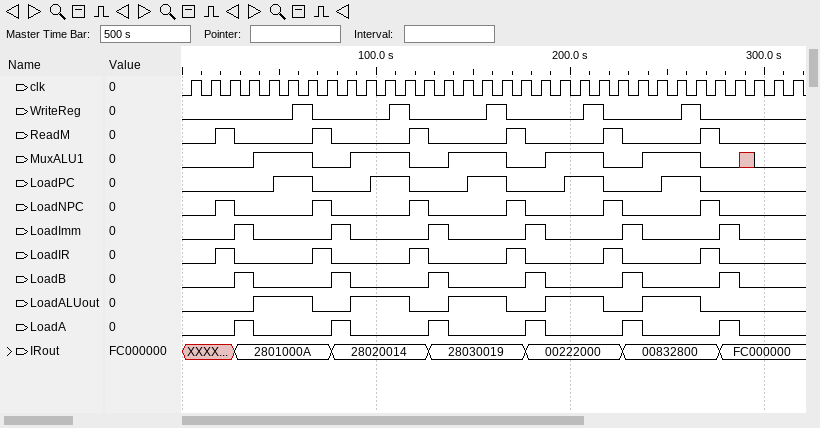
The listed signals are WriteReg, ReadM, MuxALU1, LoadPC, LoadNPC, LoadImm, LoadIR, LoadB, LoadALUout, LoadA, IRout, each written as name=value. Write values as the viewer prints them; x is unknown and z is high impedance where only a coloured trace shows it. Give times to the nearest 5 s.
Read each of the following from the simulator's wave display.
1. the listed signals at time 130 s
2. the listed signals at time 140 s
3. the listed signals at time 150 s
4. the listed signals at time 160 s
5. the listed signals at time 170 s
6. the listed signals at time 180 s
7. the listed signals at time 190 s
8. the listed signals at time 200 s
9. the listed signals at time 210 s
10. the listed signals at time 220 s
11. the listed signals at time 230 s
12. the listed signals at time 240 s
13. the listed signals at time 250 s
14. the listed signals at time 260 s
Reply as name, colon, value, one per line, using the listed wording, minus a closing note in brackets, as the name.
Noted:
the listed signals at time 130 s: WriteReg=0, ReadM=0, MuxALU1=0, LoadPC=0, LoadNPC=0, LoadImm=1, LoadIR=0, LoadB=1, LoadALUout=0, LoadA=1, IRout=28030019
the listed signals at time 140 s: WriteReg=0, ReadM=0, MuxALU1=1, LoadPC=0, LoadNPC=0, LoadImm=0, LoadIR=0, LoadB=0, LoadALUout=1, LoadA=0, IRout=28030019
the listed signals at time 150 s: WriteReg=0, ReadM=0, MuxALU1=1, LoadPC=1, LoadNPC=0, LoadImm=0, LoadIR=0, LoadB=0, LoadALUout=1, LoadA=0, IRout=28030019
the listed signals at time 160 s: WriteReg=1, ReadM=0, MuxALU1=1, LoadPC=1, LoadNPC=0, LoadImm=0, LoadIR=0, LoadB=0, LoadALUout=1, LoadA=0, IRout=28030019
the listed signals at time 170 s: WriteReg=0, ReadM=1, MuxALU1=0, LoadPC=0, LoadNPC=1, LoadImm=0, LoadIR=1, LoadB=0, LoadALUout=0, LoadA=0, IRout=28030019
the listed signals at time 180 s: WriteReg=0, ReadM=0, MuxALU1=0, LoadPC=0, LoadNPC=0, LoadImm=1, LoadIR=0, LoadB=1, LoadALUout=0, LoadA=1, IRout=00222000
the listed signals at time 190 s: WriteReg=0, ReadM=0, MuxALU1=1, LoadPC=0, LoadNPC=0, LoadImm=0, LoadIR=0, LoadB=0, LoadALUout=1, LoadA=0, IRout=00222000
the listed signals at time 200 s: WriteReg=0, ReadM=0, MuxALU1=1, LoadPC=1, LoadNPC=0, LoadImm=0, LoadIR=0, LoadB=0, LoadALUout=1, LoadA=0, IRout=00222000
the listed signals at time 210 s: WriteReg=1, ReadM=0, MuxALU1=1, LoadPC=1, LoadNPC=0, LoadImm=0, LoadIR=0, LoadB=0, LoadALUout=1, LoadA=0, IRout=00222000
the listed signals at time 220 s: WriteReg=0, ReadM=1, MuxALU1=0, LoadPC=0, LoadNPC=1, LoadImm=0, LoadIR=1, LoadB=0, LoadALUout=0, LoadA=0, IRout=00222000
the listed signals at time 230 s: WriteReg=0, ReadM=0, MuxALU1=0, LoadPC=0, LoadNPC=0, LoadImm=1, LoadIR=0, LoadB=1, LoadALUout=0, LoadA=1, IRout=00832800
the listed signals at time 240 s: WriteReg=0, ReadM=0, MuxALU1=1, LoadPC=0, LoadNPC=0, LoadImm=0, LoadIR=0, LoadB=0, LoadALUout=1, LoadA=0, IRout=00832800
the listed signals at time 250 s: WriteReg=0, ReadM=0, MuxALU1=1, LoadPC=1, LoadNPC=0, LoadImm=0, LoadIR=0, LoadB=0, LoadALUout=1, LoadA=0, IRout=00832800
the listed signals at time 260 s: WriteReg=1, ReadM=0, MuxALU1=1, LoadPC=1, LoadNPC=0, LoadImm=0, LoadIR=0, LoadB=0, LoadALUout=1, LoadA=0, IRout=00832800
